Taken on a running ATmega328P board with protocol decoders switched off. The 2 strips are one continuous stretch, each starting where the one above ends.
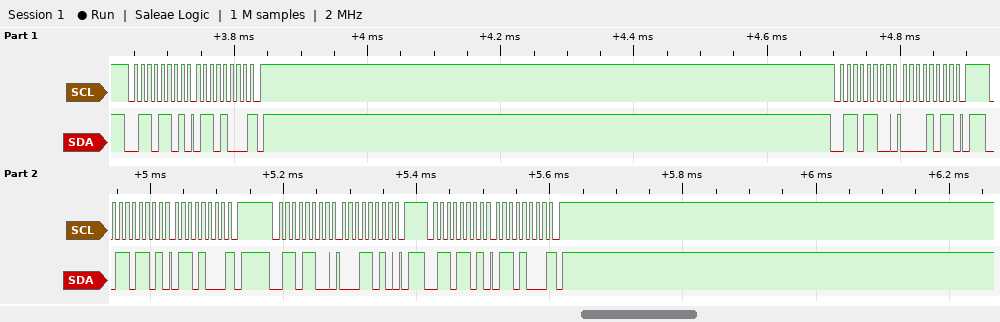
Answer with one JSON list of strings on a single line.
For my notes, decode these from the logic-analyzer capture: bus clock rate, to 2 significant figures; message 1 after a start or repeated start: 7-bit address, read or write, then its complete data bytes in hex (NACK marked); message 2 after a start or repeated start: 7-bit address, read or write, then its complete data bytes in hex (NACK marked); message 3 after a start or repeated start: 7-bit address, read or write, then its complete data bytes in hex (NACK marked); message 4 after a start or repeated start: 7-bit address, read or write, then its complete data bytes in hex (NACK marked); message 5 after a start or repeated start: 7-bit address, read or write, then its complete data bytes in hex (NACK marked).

["100 kHz", "0x36 read: 68 NACK", "0x36 write: 0B", "0x36 read: 68 NACK", "0x36 write: 1A", "0x36 read: 68 NACK"]
